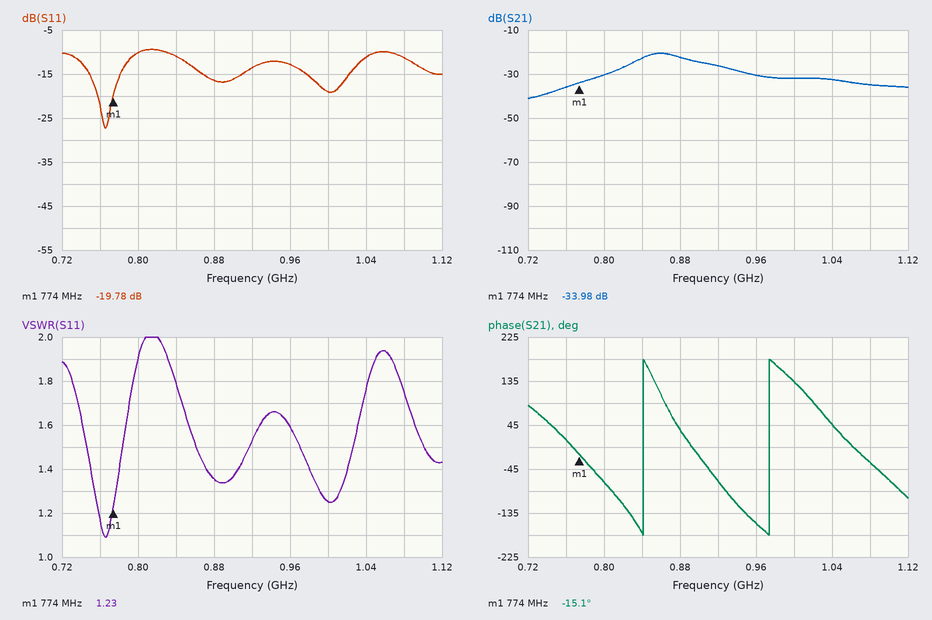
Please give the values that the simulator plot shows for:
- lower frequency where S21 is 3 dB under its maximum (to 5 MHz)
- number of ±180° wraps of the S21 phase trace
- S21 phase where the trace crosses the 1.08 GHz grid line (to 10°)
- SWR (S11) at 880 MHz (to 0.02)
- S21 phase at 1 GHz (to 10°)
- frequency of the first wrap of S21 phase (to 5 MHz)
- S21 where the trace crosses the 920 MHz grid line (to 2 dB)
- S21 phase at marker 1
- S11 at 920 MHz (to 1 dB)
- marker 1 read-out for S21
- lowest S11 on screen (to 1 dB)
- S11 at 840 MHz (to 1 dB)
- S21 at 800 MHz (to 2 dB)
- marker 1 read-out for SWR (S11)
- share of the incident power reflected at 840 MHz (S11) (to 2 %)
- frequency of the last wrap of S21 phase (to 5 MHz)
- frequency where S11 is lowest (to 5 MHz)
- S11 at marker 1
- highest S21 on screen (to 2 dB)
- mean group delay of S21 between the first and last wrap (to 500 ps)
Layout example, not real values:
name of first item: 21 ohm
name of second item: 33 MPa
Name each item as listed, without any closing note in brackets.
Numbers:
lower frequency where S21 is 3 dB under its maximum: 835 MHz
number of ±180° wraps of the S21 phase trace: 2
S21 phase where the trace crosses the 1.08 GHz grid line: -30°
SWR (S11) at 880 MHz: 1.36
S21 phase at 1 GHz: 130°
frequency of the first wrap of S21 phase: 840 MHz
S21 where the trace crosses the 920 MHz grid line: -26 dB
S21 phase at marker 1: -15.1°
S11 at 920 MHz: -14 dB
marker 1 read-out for S21: -33.98 dB
lowest S11 on screen: -27 dB
S11 at 840 MHz: -11 dB
S21 at 800 MHz: -30 dB
marker 1 read-out for SWR: 1.23
share of the incident power reflected at 840 MHz (S11): 8 %
frequency of the last wrap of S21 phase: 975 MHz
frequency where S11 is lowest: 765 MHz
S11 at marker 1: -19.78 dB
highest S21 on screen: -20 dB
mean group delay of S21 between the first and last wrap: 7.5 ns
